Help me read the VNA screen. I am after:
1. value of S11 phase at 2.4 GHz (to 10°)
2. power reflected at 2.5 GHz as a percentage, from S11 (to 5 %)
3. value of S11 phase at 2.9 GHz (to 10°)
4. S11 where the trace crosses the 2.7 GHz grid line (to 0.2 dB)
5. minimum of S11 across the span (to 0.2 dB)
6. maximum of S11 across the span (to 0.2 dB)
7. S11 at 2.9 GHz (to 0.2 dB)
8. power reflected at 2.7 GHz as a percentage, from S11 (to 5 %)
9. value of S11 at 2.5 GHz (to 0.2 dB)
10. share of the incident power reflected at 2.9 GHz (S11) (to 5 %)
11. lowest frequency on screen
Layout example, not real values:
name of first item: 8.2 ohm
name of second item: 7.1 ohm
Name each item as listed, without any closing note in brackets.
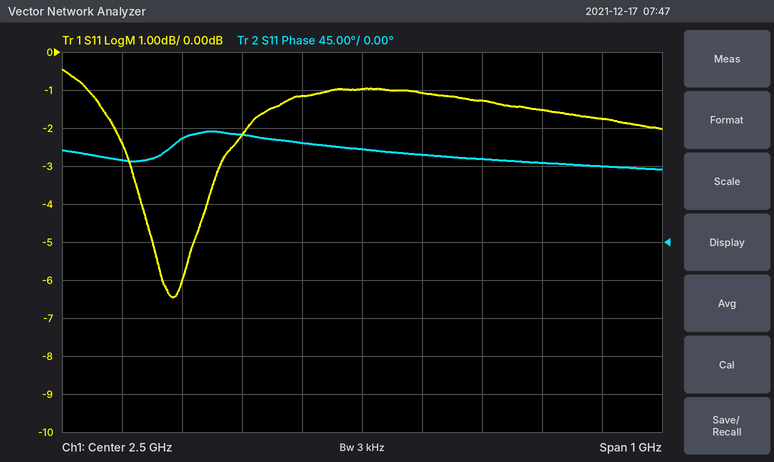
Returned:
value of S11 phase at 2.4 GHz: 120°
power reflected at 2.5 GHz as a percentage, from S11: 80 %
value of S11 phase at 2.9 GHz: 90°
S11 where the trace crosses the 2.7 GHz grid line: -1.2 dB
minimum of S11 across the span: -6.4 dB
maximum of S11 across the span: -0.4 dB
S11 at 2.9 GHz: -1.8 dB
power reflected at 2.7 GHz as a percentage, from S11: 75 %
value of S11 at 2.5 GHz: -1.0 dB
share of the incident power reflected at 2.9 GHz (S11): 65 %
lowest frequency on screen: 2 GHz
